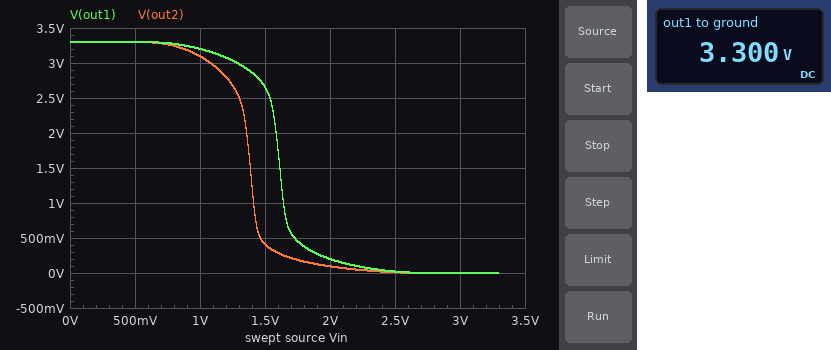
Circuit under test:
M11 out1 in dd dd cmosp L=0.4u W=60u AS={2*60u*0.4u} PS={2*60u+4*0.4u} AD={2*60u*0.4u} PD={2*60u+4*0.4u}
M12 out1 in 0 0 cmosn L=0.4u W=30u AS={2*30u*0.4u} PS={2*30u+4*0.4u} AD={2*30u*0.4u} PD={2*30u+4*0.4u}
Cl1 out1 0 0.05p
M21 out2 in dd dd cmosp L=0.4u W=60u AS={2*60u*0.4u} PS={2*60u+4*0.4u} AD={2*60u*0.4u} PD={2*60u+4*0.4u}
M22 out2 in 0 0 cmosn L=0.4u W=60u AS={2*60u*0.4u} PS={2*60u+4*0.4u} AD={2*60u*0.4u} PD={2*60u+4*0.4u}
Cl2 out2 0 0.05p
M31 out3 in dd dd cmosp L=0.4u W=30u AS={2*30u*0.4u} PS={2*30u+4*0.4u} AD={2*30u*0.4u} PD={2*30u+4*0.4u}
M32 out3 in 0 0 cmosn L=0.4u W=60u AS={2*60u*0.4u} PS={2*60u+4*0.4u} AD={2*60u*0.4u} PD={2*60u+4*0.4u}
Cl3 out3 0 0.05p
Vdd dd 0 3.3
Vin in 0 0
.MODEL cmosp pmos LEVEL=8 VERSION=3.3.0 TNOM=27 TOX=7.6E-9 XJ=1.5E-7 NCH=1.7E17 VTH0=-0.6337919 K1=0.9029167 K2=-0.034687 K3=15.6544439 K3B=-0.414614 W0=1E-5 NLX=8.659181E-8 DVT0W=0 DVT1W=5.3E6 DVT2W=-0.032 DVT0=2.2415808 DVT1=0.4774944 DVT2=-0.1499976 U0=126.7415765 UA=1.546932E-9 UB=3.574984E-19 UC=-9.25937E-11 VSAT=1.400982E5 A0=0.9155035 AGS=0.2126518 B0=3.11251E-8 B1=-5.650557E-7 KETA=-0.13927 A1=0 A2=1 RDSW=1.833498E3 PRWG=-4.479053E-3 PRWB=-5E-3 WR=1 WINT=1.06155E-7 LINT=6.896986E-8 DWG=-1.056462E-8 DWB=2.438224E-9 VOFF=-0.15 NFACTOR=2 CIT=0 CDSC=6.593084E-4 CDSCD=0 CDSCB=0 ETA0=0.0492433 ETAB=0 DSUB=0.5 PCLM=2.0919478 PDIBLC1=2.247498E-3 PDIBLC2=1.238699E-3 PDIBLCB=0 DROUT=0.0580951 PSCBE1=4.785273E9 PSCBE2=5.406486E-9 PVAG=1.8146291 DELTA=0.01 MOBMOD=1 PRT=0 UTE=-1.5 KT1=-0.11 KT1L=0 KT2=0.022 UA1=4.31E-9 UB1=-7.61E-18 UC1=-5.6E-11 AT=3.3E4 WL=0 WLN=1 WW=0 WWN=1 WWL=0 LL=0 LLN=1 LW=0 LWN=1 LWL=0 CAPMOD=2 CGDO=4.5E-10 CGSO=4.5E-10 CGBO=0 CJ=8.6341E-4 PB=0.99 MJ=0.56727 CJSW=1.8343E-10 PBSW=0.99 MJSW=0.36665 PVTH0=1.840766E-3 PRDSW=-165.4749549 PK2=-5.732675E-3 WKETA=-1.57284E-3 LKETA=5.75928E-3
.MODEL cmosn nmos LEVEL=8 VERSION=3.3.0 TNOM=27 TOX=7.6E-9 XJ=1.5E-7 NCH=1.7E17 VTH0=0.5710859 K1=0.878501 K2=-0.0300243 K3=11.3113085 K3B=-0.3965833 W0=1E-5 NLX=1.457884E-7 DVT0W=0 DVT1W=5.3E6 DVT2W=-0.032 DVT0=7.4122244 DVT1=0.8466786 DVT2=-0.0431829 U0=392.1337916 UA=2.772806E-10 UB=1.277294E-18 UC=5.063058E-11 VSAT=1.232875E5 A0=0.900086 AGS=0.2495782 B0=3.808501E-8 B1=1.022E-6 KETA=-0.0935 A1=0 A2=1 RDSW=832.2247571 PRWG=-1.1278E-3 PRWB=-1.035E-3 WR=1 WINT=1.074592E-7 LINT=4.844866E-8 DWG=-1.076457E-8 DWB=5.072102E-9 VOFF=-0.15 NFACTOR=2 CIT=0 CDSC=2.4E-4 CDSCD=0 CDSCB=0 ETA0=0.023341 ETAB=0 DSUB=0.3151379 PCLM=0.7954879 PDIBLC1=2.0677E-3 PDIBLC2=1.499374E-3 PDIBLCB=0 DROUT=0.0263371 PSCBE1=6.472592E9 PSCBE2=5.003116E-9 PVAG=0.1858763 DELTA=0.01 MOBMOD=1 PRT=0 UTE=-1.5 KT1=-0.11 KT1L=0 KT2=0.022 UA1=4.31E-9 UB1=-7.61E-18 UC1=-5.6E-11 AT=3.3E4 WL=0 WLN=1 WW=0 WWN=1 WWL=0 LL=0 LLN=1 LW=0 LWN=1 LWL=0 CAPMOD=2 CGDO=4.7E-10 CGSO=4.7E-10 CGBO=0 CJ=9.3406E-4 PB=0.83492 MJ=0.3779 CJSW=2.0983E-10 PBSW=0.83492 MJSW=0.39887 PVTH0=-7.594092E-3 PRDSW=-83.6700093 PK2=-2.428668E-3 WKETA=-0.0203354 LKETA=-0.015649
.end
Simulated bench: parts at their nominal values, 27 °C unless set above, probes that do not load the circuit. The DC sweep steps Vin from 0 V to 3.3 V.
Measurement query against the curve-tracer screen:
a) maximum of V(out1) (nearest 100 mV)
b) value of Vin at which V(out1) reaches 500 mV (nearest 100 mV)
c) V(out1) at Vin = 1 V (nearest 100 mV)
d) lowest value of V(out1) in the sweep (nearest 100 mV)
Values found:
3.3 V
1.7 V
3.2 V
0 V
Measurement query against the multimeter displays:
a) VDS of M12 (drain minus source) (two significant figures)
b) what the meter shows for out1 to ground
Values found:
3.3 V
3.300 V
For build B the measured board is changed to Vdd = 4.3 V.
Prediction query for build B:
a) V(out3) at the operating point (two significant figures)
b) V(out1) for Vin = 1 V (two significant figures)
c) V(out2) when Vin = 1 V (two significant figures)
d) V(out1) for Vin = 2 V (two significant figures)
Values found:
4.3 V
4.2 V
4.1 V
3.2 V
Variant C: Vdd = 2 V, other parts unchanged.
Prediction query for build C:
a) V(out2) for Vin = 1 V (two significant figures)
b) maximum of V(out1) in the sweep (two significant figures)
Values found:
110 mV
2.0 V
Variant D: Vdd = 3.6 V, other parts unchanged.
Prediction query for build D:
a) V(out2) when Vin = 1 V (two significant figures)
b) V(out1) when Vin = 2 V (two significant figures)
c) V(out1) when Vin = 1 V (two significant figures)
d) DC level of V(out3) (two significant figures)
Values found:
3.4 V
400 mV
3.5 V
3.6 V
